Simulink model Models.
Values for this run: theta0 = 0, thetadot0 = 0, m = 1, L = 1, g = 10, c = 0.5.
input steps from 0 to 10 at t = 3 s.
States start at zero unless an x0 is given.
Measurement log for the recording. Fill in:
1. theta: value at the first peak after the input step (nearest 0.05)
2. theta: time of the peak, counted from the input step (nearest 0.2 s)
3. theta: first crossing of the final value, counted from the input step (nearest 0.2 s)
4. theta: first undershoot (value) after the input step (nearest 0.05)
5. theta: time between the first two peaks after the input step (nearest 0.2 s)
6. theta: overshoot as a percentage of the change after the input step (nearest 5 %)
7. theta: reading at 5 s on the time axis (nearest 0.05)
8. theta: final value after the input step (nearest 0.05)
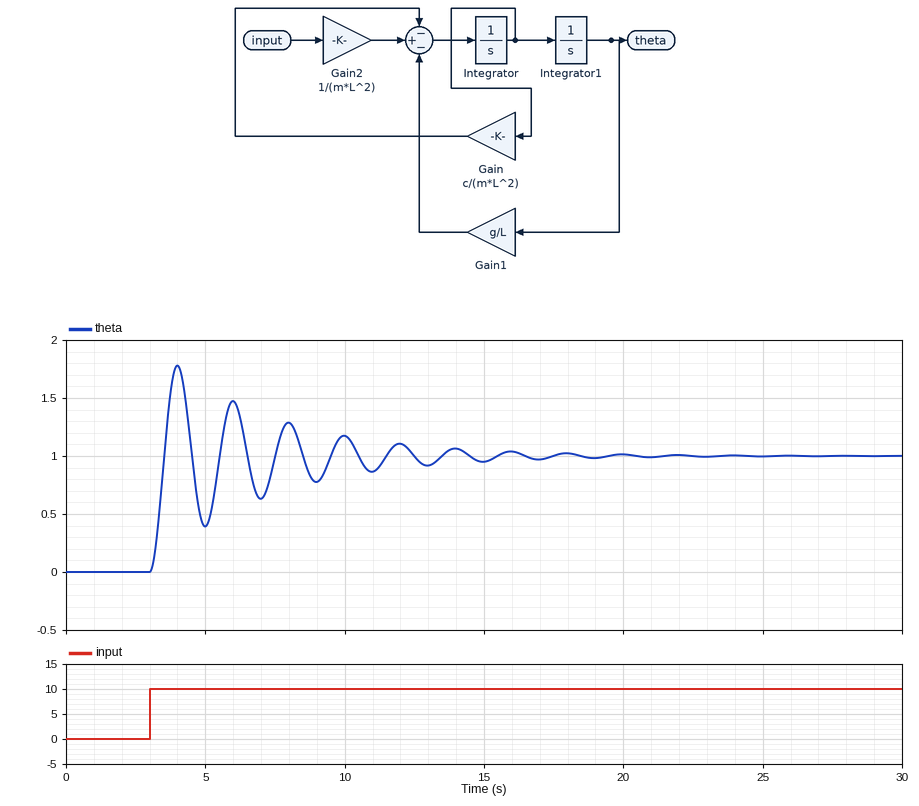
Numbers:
1.80
1.0 s
0.6 s
0.40
2.0 s
80 %
0.40
1.00
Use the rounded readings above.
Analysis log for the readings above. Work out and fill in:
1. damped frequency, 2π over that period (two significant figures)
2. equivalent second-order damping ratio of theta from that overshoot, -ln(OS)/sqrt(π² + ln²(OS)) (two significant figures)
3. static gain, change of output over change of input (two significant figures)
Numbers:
3.1 rad/s
0.071
0.10
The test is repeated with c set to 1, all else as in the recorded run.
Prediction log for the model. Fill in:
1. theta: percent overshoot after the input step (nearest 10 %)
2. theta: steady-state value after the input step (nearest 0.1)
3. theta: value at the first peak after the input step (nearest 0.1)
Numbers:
60 %
1.0
1.6
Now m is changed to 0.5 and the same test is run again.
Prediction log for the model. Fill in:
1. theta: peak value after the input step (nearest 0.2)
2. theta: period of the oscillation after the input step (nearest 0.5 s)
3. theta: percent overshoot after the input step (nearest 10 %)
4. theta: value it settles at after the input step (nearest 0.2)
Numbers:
3.2
2.0 s
60 %
2.0
